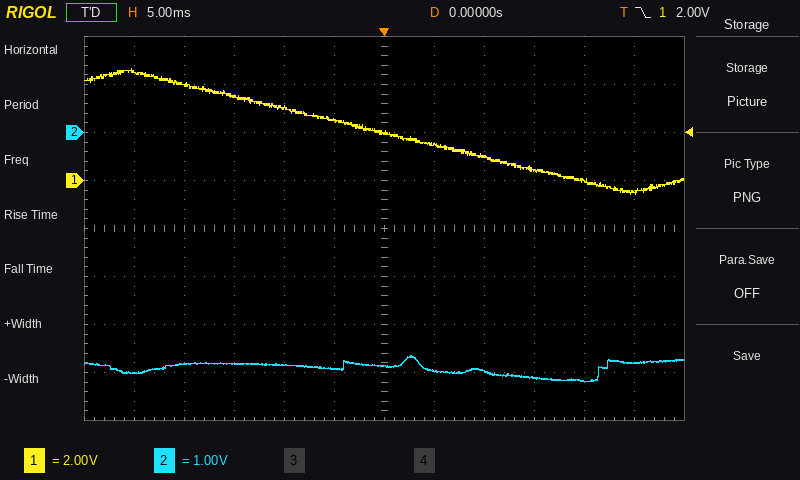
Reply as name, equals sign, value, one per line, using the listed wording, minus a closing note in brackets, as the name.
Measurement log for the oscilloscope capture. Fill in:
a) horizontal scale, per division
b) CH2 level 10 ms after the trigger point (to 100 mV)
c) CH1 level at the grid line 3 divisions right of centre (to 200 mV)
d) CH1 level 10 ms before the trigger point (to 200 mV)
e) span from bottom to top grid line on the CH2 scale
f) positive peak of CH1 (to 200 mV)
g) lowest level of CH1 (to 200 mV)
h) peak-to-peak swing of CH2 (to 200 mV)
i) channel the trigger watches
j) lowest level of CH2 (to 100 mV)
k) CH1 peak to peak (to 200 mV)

horizontal scale, per division = 5 ms
CH2 level 10 ms after the trigger point = -5.0 V
CH1 level at the grid line 3 divisions right of centre = 400 mV
CH1 level 10 ms before the trigger point = 3.0 V
span from bottom to top grid line on the CH2 scale = 8 V
positive peak of CH1 = 4.6 V
lowest level of CH1 = -600 mV
peak-to-peak swing of CH2 = 600 mV
channel the trigger watches = CH1
lowest level of CH2 = -5.2 V
CH1 peak to peak = 5.2 V
